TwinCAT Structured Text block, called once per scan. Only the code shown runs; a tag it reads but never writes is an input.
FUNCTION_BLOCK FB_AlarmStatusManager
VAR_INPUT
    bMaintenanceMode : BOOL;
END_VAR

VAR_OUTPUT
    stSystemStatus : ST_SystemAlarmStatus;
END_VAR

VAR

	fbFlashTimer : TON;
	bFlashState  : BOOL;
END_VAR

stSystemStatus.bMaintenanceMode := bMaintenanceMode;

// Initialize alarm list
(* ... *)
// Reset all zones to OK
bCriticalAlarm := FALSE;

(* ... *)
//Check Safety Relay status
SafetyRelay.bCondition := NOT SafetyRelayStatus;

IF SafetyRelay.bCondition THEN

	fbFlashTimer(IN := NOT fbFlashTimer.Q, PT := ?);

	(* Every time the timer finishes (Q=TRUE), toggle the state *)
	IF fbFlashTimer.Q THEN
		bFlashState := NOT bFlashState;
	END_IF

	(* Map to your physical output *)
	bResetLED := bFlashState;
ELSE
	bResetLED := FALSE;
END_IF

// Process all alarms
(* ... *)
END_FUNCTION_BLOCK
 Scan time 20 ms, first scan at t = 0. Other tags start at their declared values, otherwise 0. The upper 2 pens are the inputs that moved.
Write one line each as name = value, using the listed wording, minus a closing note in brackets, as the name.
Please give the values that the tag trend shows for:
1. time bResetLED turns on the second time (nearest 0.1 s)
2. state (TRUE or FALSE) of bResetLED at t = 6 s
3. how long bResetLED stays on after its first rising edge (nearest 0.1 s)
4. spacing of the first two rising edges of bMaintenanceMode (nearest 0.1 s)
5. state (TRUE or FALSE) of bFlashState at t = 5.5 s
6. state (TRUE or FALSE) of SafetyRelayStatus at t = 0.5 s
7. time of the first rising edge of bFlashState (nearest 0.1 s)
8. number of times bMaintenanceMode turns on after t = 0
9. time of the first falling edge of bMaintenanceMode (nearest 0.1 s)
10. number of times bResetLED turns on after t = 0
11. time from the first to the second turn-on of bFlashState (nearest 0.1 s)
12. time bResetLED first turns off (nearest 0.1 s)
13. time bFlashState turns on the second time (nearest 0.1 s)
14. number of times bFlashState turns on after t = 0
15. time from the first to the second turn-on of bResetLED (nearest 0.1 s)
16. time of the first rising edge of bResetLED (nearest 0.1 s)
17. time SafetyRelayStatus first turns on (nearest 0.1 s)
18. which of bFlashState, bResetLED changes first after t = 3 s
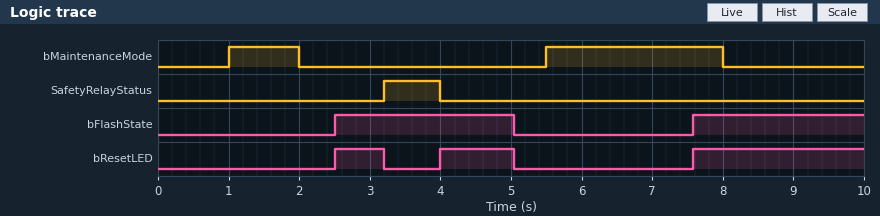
time bResetLED turns on the second time = 4.0 s
state (TRUE or FALSE) of bResetLED at t = 6 s = FALSE
how long bResetLED stays on after its first rising edge = 0.7 s
spacing of the first two rising edges of bMaintenanceMode = 4.5 s
state (TRUE or FALSE) of bFlashState at t = 5.5 s = FALSE
state (TRUE or FALSE) of SafetyRelayStatus at t = 0.5 s = FALSE
time of the first rising edge of bFlashState = 2.5 s
number of times bMaintenanceMode turns on after t = 0 = 2
time of the first falling edge of bMaintenanceMode = 2.0 s
number of times bResetLED turns on after t = 0 = 3
time from the first to the second turn-on of bFlashState = 5.1 s
time bResetLED first turns off = 3.2 s
time bFlashState turns on the second time = 7.6 s
number of times bFlashState turns on after t = 0 = 2
time from the first to the second turn-on of bResetLED = 1.5 s
time of the first rising edge of bResetLED = 2.5 s
time SafetyRelayStatus first turns on = 3.2 s
which of bFlashState, bResetLED changes first after t = 3 s = bResetLED
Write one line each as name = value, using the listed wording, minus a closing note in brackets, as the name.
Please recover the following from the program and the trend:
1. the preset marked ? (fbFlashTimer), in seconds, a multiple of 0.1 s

the preset marked ? (fbFlashTimer), in seconds, a multiple of 0.1 s = 2.5 s
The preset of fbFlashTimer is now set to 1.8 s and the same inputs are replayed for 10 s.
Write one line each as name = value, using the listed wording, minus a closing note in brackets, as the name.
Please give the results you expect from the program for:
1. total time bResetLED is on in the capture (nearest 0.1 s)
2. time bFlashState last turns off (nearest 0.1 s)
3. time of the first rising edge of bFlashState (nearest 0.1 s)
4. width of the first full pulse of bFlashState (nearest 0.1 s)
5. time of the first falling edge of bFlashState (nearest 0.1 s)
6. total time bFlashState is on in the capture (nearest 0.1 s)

total time bResetLED is on in the capture = 3.7 s
time bFlashState last turns off = 7.7 s
time of the first rising edge of bFlashState = 1.8 s
width of the first full pulse of bFlashState = 2.2 s
time of the first falling edge of bFlashState = 4.0 s
total time bFlashState is on in the capture = 4.5 s
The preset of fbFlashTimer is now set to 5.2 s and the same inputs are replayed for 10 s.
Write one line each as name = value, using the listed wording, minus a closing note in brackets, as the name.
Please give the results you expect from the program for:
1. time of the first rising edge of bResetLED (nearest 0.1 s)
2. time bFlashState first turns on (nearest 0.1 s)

time of the first rising edge of bResetLED = 5.2 s
time bFlashState first turns on = 5.2 s
